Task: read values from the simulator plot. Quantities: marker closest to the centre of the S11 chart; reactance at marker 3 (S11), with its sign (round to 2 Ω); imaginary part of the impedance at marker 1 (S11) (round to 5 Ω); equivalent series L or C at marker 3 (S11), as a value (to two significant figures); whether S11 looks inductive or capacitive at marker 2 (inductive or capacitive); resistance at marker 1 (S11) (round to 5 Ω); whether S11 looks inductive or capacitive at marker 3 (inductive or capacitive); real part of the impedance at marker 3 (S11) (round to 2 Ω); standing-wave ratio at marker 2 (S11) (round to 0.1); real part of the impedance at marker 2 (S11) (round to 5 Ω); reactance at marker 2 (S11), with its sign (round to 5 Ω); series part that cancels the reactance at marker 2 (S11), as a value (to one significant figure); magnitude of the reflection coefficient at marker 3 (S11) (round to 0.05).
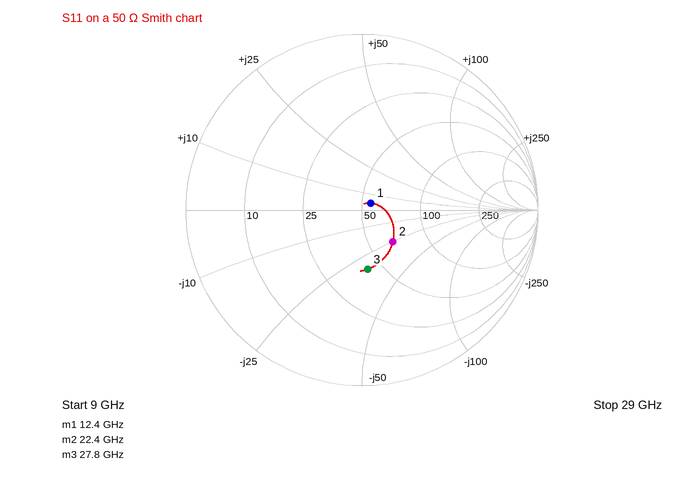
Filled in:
marker 1
-32 Ω
+5 Ω
180 fF
capacitive
55 Ω
capacitive
42 Ω
1.7
65 Ω
-25 Ω
200 pH
0.35
